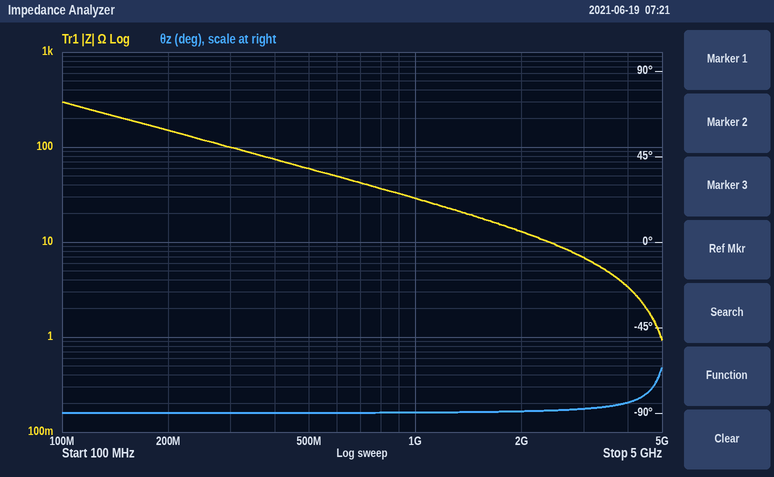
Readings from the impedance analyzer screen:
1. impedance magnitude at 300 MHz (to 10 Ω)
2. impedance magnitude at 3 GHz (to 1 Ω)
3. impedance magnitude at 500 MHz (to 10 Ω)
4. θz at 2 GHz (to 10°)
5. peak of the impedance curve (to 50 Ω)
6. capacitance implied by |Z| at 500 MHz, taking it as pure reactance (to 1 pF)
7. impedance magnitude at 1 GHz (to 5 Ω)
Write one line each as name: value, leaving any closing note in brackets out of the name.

impedance magnitude at 300 MHz: 100 Ω
impedance magnitude at 3 GHz: 7 Ω
impedance magnitude at 500 MHz: 60 Ω
θz at 2 GHz: -90°
peak of the impedance curve: 300 Ω
capacitance implied by |Z| at 500 MHz, taking it as pure reactance: 5 pF
impedance magnitude at 1 GHz: 30 Ω
